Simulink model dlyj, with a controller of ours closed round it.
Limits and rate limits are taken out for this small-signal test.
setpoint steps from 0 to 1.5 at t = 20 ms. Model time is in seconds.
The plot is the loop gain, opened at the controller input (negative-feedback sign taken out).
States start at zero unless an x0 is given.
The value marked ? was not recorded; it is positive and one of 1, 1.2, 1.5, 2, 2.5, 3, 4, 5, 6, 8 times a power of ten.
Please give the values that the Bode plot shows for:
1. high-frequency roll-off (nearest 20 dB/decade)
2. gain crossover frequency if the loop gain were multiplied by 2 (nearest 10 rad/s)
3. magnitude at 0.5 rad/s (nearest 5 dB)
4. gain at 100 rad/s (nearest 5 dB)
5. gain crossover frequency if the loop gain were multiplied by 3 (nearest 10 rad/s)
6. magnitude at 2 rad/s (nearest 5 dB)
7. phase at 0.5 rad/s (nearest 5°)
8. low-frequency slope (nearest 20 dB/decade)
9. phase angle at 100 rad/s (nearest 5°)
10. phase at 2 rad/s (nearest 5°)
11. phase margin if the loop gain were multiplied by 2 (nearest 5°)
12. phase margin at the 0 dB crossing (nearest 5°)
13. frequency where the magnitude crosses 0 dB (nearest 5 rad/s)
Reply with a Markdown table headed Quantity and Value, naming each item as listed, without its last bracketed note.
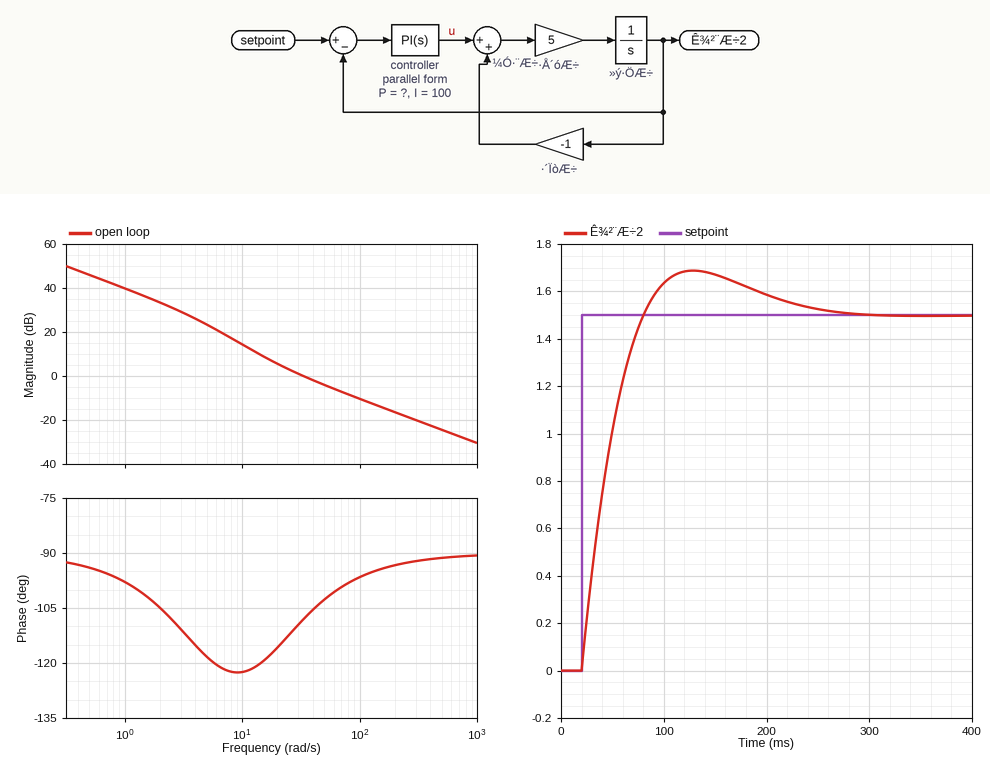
| Quantity | Value |
|---|---|
| high-frequency roll-off | -20 dB/decade |
| gain crossover frequency if the loop gain were multiplied by 2 | 60 rad/s |
| magnitude at 0.5 rad/s | 45 dB |
| gain at 100 rad/s | -10 dB |
| gain crossover frequency if the loop gain were multiplied by 3 | 90 rad/s |
| magnitude at 2 rad/s | 35 dB |
| phase at 0.5 rad/s | -95° |
| low-frequency slope | -20 dB/decade |
| phase angle at 100 rad/s | -95° |
| phase at 2 rad/s | -105° |
| phase margin if the loop gain were multiplied by 2 | 80° |
| phase margin at the 0 dB crossing | 70° |
| frequency where the magnitude crosses 0 dB | 35 rad/s |
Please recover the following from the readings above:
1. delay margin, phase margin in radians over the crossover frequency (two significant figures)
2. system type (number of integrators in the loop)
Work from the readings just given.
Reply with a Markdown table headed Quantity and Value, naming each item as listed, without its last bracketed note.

| Quantity | Value |
|---|---|
| delay margin, phase margin in radians over the crossover frequency | 0.035 s |
| system type | 1 |
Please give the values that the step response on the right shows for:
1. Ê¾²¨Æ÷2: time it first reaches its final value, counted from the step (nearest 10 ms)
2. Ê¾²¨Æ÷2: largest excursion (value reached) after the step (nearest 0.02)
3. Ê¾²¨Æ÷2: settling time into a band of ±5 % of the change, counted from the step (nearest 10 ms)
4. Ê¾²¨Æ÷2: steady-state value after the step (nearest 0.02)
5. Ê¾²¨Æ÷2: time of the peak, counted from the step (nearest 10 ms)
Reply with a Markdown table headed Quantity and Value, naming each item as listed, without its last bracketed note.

| Quantity | Value |
|---|---|
| Ê¾²¨Æ÷2: time it first reaches its final value, counted from the step | 60 ms |
| Ê¾²¨Æ÷2: largest excursion (value reached) after the step | 1.68 |
| Ê¾²¨Æ÷2: settling time into a band of ±5 % of the change, counted from the step | 190 ms |
| Ê¾²¨Æ÷2: steady-state value after the step | 1.50 |
| Ê¾²¨Æ÷2: time of the peak, counted from the step | 110 ms |
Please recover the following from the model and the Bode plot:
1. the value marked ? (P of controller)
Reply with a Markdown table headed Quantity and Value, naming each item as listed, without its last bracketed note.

| Quantity | Value |
|---|---|
| the value marked ? | 6 |
